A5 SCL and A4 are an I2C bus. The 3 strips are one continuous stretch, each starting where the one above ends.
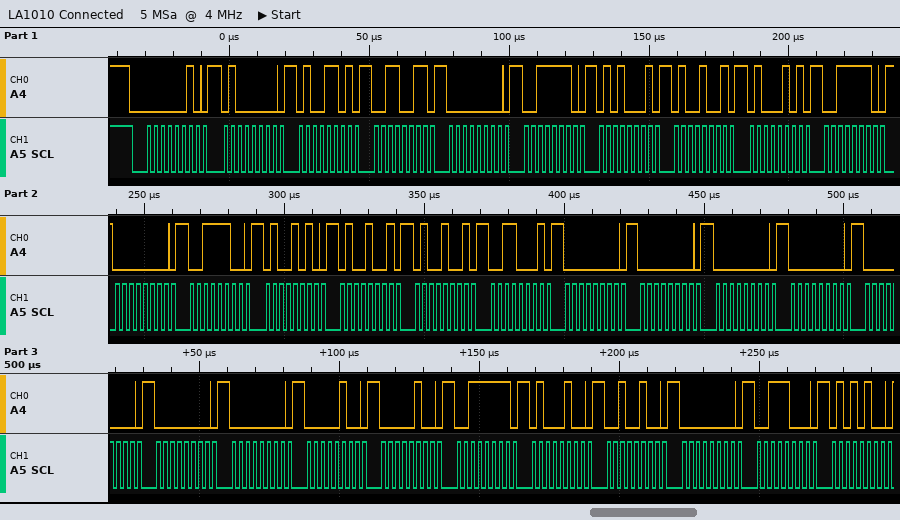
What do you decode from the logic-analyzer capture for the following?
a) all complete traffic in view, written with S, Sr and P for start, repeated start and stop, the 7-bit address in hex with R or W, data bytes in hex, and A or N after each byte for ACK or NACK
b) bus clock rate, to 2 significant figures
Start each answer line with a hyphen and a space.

- S 01W A 40 A 4D A 33 A 00 A 3E A 51 A 49 A 45 A 3E A 00 A 3C A 4A A 49 A 49 A 31 A 00 A 00 A 00 A 00 A 00 A 00 A 00 A 04 A 04 A 3F A 44 A 24 A 00 A 38 A 54 A
- 400 kHz
